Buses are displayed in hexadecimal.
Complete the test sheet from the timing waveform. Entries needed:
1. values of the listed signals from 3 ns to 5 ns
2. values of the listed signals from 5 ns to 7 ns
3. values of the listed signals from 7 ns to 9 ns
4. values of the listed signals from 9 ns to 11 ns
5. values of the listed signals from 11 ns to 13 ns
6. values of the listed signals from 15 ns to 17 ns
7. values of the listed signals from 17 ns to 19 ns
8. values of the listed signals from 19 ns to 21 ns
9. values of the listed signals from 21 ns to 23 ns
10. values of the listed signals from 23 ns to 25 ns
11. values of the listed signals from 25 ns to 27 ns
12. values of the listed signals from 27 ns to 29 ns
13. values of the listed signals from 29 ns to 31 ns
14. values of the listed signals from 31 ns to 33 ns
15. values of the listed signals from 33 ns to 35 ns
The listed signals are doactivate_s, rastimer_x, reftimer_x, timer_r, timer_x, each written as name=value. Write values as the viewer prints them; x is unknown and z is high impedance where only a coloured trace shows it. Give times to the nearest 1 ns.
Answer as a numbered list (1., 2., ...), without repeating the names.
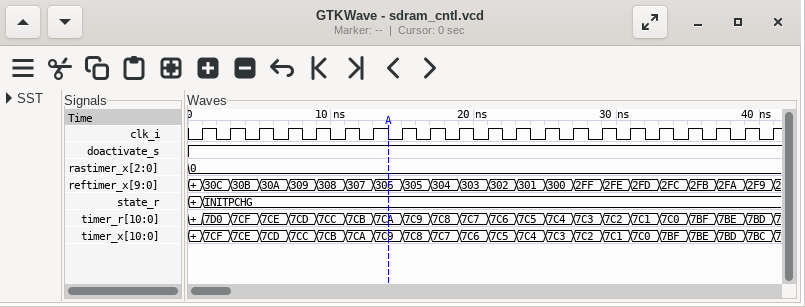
1. doactivate_s=1, rastimer_x=0, reftimer_x=30B, timer_r=7CF, timer_x=7CE
2. doactivate_s=1, rastimer_x=0, reftimer_x=30A, timer_r=7CE, timer_x=7CD
3. doactivate_s=1, rastimer_x=0, reftimer_x=309, timer_r=7CD, timer_x=7CC
4. doactivate_s=1, rastimer_x=0, reftimer_x=308, timer_r=7CC, timer_x=7CB
5. doactivate_s=1, rastimer_x=0, reftimer_x=307, timer_r=7CB, timer_x=7CA
6. doactivate_s=1, rastimer_x=0, reftimer_x=305, timer_r=7C9, timer_x=7C8
7. doactivate_s=1, rastimer_x=0, reftimer_x=304, timer_r=7C8, timer_x=7C7
8. doactivate_s=1, rastimer_x=0, reftimer_x=303, timer_r=7C7, timer_x=7C6
9. doactivate_s=1, rastimer_x=0, reftimer_x=302, timer_r=7C6, timer_x=7C5
10. doactivate_s=1, rastimer_x=0, reftimer_x=301, timer_r=7C5, timer_x=7C4
11. doactivate_s=1, rastimer_x=0, reftimer_x=300, timer_r=7C4, timer_x=7C3
12. doactivate_s=1, rastimer_x=0, reftimer_x=2FF, timer_r=7C3, timer_x=7C2
13. doactivate_s=1, rastimer_x=0, reftimer_x=2FE, timer_r=7C2, timer_x=7C1
14. doactivate_s=1, rastimer_x=0, reftimer_x=2FD, timer_r=7C1, timer_x=7C0
15. doactivate_s=1, rastimer_x=0, reftimer_x=2FC, timer_r=7C0, timer_x=7BF
